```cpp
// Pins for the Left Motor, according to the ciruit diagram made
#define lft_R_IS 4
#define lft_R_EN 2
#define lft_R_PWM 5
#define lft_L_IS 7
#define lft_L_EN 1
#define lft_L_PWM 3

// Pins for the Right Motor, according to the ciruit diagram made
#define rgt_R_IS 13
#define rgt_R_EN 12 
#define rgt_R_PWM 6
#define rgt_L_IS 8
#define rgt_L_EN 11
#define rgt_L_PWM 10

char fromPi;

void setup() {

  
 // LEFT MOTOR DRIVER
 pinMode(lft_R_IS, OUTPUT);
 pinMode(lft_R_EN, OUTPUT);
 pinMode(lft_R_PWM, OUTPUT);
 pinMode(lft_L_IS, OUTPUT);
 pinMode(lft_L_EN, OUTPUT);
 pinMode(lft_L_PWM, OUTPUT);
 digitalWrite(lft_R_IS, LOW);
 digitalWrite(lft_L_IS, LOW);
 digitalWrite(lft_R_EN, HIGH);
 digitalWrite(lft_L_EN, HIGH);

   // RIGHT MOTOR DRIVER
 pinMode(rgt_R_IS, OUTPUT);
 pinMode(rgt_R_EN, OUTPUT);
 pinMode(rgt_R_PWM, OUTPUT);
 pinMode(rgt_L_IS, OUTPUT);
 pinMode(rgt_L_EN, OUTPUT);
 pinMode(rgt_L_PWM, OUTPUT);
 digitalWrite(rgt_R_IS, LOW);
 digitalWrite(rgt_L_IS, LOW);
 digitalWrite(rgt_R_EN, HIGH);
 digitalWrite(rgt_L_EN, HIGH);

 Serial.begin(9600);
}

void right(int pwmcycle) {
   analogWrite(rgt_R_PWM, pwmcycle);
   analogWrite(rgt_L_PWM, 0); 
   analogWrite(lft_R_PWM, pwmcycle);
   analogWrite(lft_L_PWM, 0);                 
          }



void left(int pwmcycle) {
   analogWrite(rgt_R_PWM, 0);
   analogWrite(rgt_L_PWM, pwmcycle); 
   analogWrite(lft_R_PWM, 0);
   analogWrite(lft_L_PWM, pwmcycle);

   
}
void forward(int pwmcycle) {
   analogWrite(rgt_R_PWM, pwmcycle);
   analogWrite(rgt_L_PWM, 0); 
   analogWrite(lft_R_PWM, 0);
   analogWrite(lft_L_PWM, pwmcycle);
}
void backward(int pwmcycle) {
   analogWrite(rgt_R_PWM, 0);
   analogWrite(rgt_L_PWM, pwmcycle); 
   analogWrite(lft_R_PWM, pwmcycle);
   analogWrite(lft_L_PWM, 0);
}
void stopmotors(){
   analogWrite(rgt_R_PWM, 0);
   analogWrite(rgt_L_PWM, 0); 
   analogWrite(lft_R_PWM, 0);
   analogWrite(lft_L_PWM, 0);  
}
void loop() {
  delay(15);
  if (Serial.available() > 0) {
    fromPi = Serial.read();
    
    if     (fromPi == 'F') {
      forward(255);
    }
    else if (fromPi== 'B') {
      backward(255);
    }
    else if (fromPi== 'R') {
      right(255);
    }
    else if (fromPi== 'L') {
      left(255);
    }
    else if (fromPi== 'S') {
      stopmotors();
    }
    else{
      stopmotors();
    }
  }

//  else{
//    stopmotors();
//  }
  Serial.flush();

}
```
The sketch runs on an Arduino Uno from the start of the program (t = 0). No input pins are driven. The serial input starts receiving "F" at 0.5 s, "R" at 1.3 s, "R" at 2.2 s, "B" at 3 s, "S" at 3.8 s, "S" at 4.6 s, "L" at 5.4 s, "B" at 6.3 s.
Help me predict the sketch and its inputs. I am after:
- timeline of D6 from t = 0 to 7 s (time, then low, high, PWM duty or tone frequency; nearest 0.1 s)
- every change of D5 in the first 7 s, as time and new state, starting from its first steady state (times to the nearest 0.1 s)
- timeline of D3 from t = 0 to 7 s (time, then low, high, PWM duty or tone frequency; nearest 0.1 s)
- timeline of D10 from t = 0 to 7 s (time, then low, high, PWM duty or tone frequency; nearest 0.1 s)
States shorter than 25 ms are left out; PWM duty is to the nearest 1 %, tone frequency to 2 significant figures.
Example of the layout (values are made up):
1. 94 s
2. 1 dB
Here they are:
1. 0 s low; 0.5 s high; 3 s low
2. 0 s low; 1.3 s high; 3.8 s low; 6.3 s high
3. 0 s low; 0.5 s high; 1.3 s low; 5.4 s high; 6.3 s low
4. 0 s low; 3 s high; 3.8 s low; 5.4 s high
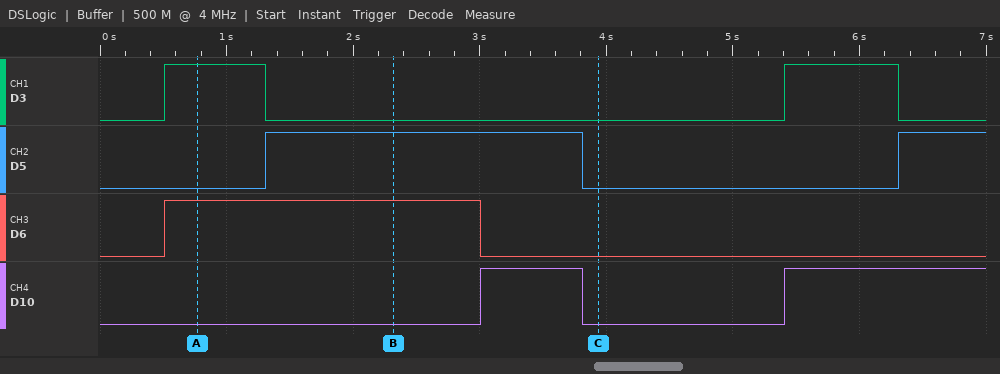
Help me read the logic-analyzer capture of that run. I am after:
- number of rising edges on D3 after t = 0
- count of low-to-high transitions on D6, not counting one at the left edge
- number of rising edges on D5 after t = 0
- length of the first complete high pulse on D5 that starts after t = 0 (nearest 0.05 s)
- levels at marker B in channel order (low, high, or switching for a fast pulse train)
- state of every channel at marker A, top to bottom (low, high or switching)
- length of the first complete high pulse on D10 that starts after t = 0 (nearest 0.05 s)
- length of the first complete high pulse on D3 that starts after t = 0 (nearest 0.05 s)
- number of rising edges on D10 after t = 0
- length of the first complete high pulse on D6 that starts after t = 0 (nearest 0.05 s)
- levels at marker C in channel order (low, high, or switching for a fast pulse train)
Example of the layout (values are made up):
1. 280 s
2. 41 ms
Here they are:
1. 2
2. 1
3. 2
4. 2.50 s
5. D3 low, D5 high, D6 high, D10 low
6. D3 high, D5 low, D6 high, D10 low
7. 0.80 s
8. 0.80 s
9. 2
10. 2.50 s
11. D3 low, D5 low, D6 low, D10 low
